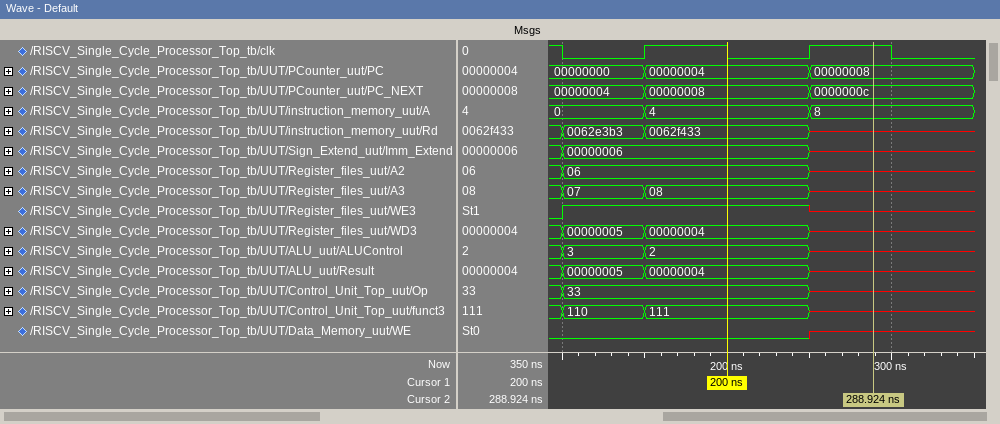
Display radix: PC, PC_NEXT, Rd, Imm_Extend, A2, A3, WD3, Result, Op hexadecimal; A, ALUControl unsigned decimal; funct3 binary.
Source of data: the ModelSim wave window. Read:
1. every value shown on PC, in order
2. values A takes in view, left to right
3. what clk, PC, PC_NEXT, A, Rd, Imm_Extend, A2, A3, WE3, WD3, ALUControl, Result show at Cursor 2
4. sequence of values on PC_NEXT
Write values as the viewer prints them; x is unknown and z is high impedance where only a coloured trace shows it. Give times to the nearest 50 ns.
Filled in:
00000000, 00000004, 00000008
0, 4, 8
clk=1, PC=00000008, PC_NEXT=0000000c, A=8, Rd=x, Imm_Extend=x, A2=x, A3=x, WE3=x, WD3=x, ALUControl=x, Result=x
00000004, 00000008, 0000000c
